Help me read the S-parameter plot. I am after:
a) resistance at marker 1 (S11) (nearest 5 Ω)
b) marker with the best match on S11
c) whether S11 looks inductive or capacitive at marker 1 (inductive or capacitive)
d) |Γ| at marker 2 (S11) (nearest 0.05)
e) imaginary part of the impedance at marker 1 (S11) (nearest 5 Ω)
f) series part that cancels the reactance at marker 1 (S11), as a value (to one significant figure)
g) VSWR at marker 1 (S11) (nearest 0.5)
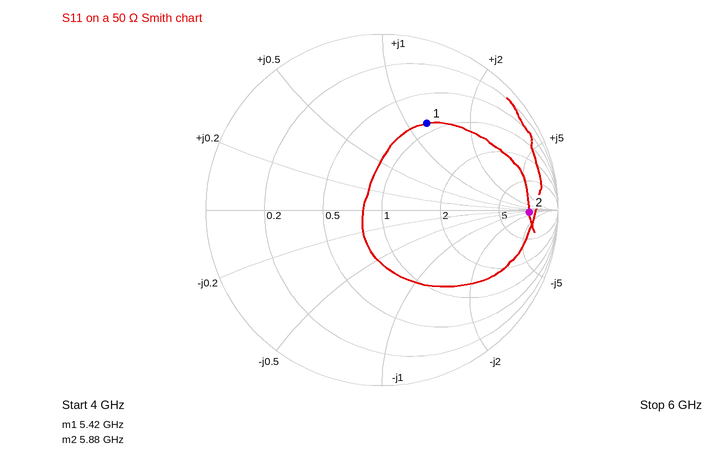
45 Ω
marker 1
inductive
0.85
+60 Ω
500 fF
3.5
